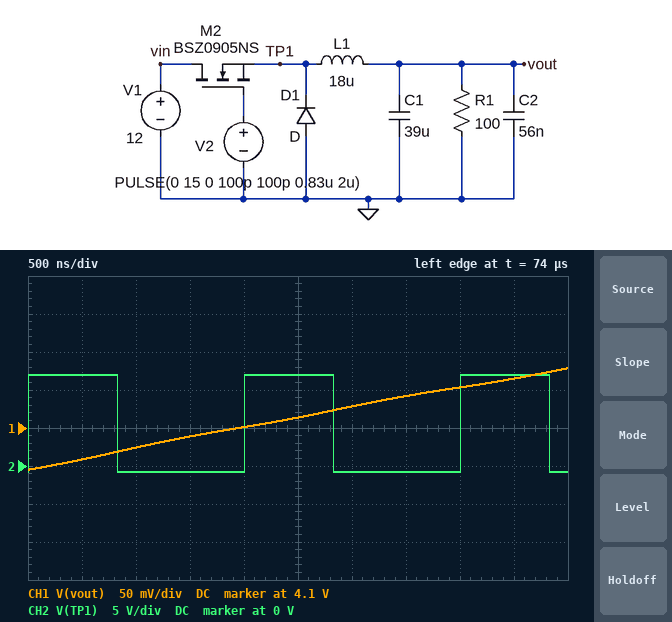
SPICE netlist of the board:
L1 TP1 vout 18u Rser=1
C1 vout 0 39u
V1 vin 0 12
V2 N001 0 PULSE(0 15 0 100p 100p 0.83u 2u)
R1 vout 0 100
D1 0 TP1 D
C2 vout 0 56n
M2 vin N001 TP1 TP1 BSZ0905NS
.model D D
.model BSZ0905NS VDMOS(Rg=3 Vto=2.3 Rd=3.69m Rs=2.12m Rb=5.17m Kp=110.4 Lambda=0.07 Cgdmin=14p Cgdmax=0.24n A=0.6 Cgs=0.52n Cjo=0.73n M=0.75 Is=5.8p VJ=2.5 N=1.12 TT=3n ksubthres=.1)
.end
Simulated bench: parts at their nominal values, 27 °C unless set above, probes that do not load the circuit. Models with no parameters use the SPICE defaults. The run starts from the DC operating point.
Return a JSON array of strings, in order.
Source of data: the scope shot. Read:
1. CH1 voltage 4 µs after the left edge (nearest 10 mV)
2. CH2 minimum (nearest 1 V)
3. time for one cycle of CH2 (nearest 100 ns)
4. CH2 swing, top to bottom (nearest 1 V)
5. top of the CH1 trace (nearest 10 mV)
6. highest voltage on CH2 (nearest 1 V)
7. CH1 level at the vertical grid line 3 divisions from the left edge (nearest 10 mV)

["4.15 V", "-1 V", "2.0 µs", "13 V", "4.18 V", "12 V", "4.09 V"]
